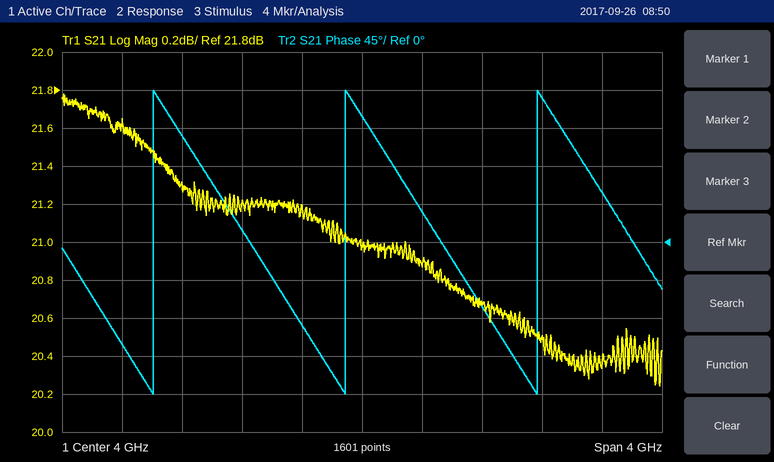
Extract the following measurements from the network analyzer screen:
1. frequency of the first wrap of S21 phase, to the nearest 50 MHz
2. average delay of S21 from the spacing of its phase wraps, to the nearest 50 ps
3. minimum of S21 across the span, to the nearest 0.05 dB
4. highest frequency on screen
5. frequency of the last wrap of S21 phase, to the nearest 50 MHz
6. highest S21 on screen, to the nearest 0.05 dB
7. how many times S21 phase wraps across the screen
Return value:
2.60 GHz
800 ps
20.25 dB
6 GHz
5.15 GHz
21.80 dB
3
